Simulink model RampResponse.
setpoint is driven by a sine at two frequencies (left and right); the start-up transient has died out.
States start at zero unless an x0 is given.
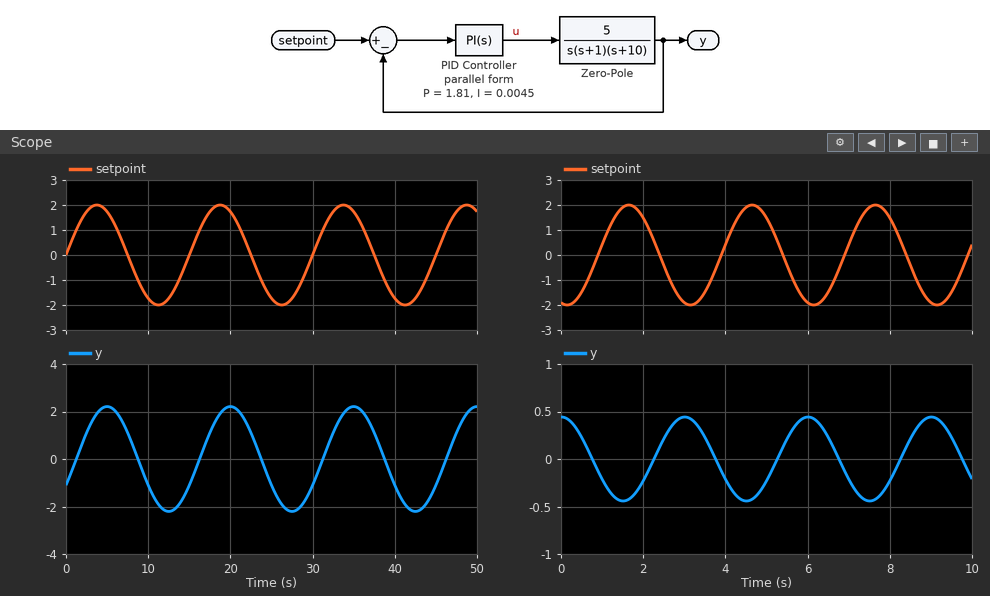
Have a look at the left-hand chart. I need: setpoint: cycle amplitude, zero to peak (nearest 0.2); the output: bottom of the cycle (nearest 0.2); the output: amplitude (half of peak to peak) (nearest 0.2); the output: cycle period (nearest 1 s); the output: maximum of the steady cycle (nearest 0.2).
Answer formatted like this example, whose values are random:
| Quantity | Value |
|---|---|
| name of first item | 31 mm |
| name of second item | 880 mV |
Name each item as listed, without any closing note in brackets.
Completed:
| Quantity | Value |
|---|---|
| setpoint: cycle amplitude, zero to peak | 2.0 |
| the output: bottom of the cycle | -2.2 |
| the output: amplitude (half of peak to peak) | 2.2 |
| the output: cycle period | 15 s |
| the output: maximum of the steady cycle | 2.2 |
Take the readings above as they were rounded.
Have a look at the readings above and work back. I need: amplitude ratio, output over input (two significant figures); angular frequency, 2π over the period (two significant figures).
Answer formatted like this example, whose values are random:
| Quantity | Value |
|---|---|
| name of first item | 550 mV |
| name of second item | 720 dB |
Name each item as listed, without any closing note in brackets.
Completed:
| Quantity | Value |
|---|---|
| amplitude ratio, output over input | 1.1 |
| angular frequency, 2π over the period | 0.42 rad/s |
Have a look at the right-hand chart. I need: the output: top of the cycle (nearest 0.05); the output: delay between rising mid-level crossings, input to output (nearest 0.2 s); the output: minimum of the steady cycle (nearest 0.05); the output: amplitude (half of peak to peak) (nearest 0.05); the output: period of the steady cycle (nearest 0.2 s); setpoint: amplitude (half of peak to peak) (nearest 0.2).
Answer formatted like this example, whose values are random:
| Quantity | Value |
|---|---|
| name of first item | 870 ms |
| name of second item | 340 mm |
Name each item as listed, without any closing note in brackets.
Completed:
| Quantity | Value |
|---|---|
| the output: top of the cycle | 0.45 |
| the output: delay between rising mid-level crossings, input to output | 1.4 s |
| the output: minimum of the steady cycle | -0.45 |
| the output: amplitude (half of peak to peak) | 0.45 |
| the output: period of the steady cycle | 3.0 s |
| setpoint: amplitude (half of peak to peak) | 2.0 |
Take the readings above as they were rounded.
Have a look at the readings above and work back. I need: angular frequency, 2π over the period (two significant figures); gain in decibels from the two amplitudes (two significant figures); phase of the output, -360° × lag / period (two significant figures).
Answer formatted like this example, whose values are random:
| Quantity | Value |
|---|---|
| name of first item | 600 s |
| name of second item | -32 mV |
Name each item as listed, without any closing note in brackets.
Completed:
| Quantity | Value |
|---|---|
| angular frequency, 2π over the period | 2.1 rad/s |
| gain in decibels from the two amplitudes | -13 dB |
| phase of the output, -360° × lag / period | -170° |
